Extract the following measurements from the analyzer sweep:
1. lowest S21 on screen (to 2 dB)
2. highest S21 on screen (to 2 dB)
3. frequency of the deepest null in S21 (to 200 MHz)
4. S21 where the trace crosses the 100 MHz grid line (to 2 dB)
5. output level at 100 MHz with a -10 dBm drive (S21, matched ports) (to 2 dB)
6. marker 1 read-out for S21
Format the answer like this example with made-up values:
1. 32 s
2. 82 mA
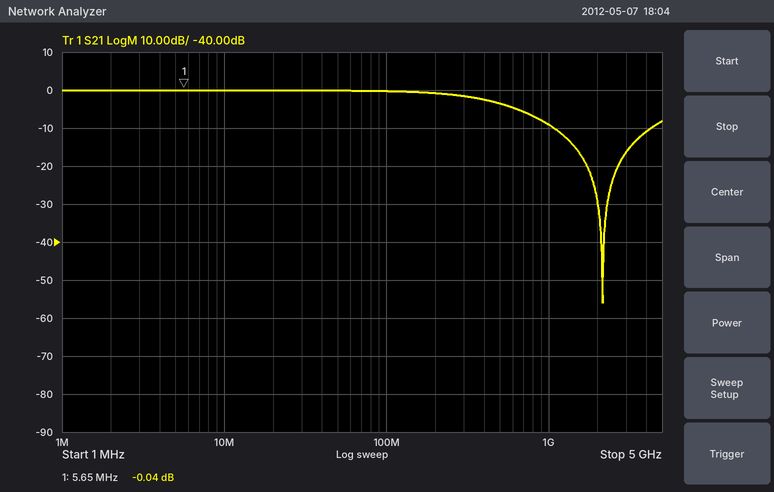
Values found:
1. -56 dB
2. 0 dB
3. 2.2 GHz
4. 0 dB
5. -10 dBm
6. -0.04 dB
